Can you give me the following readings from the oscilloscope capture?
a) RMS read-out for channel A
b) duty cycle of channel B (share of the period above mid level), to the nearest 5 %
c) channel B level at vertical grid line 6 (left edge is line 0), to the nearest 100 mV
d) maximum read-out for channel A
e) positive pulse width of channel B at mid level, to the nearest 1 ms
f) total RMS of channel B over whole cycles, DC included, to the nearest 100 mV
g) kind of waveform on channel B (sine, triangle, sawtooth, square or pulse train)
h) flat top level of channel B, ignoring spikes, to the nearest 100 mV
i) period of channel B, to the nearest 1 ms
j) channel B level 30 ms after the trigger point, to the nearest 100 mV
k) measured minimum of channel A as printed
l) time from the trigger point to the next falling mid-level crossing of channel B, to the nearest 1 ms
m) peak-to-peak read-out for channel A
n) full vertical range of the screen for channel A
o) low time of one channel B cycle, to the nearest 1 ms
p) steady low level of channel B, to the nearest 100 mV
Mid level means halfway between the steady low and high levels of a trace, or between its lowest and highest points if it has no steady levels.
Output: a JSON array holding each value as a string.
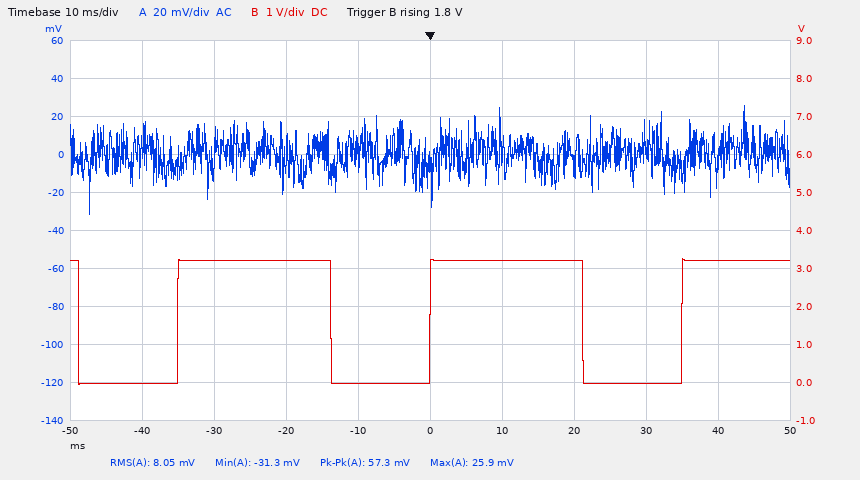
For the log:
["8.05 mV", "60 %", "3.2 V", "25.9 mV", "21 ms", "2.5 V", "pulse train", "3.2 V", "35 ms", "0.0 V", "-31.3 mV", "21 ms", "57.3 mV", "200 mV", "14 ms", "0.0 V"]
